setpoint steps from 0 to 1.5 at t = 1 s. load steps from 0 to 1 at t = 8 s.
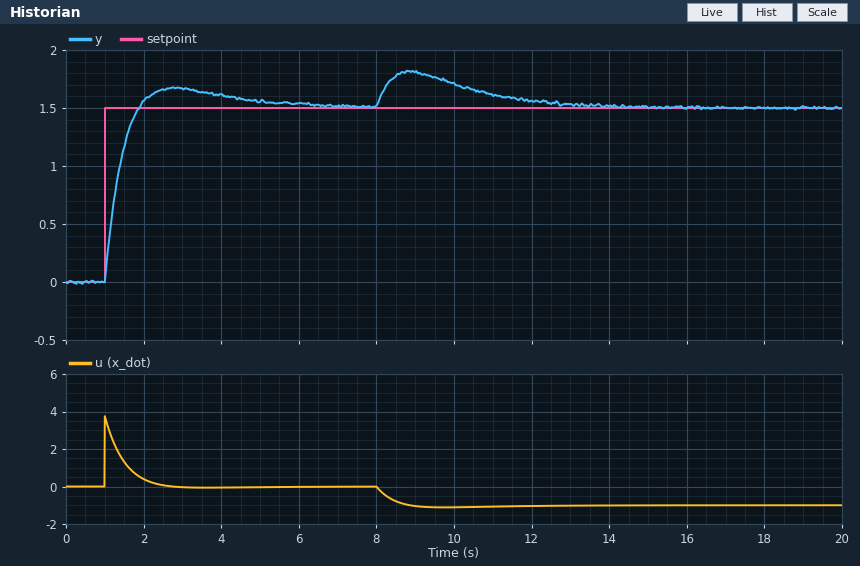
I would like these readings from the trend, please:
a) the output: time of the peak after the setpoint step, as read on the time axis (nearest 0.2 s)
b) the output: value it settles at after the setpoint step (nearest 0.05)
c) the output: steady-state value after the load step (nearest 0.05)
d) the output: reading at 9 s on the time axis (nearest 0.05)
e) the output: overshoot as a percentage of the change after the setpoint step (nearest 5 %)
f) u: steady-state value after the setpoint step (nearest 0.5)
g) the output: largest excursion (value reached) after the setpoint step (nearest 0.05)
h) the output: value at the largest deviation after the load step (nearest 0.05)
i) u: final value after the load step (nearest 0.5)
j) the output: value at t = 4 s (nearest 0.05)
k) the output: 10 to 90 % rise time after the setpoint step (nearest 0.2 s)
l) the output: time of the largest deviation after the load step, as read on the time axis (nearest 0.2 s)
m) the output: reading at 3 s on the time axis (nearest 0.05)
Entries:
2.8 s
1.50
1.50
1.80
10 %
0.0
1.65
1.80
-1.0
1.60
0.6 s
8.8 s
1.65
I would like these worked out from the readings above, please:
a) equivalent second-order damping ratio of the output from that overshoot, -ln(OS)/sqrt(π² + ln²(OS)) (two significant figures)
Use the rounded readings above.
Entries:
0.59
